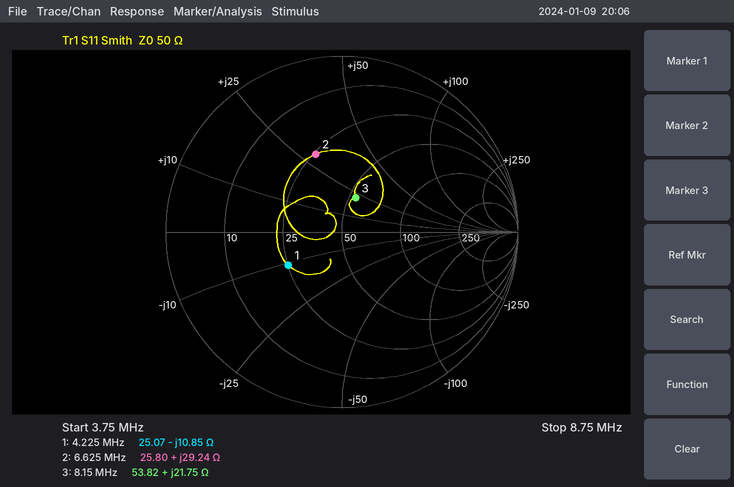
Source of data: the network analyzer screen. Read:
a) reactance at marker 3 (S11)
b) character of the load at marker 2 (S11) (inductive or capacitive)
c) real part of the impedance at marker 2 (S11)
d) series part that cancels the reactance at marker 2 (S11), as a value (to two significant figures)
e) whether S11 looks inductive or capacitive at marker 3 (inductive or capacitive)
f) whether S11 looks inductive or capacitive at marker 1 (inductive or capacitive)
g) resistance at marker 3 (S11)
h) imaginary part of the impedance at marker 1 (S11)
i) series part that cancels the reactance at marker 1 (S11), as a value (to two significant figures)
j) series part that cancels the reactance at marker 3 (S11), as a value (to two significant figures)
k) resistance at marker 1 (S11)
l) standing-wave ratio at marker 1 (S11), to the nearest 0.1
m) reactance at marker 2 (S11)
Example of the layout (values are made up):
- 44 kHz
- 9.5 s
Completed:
- +21.75 Ω
- inductive
- 25.80 Ω
- 820 pF
- inductive
- capacitive
- 53.82 Ω
- -10.85 Ω
- 410 nH
- 900 pF
- 25.07 Ω
- 2.1
- +29.24 Ω
